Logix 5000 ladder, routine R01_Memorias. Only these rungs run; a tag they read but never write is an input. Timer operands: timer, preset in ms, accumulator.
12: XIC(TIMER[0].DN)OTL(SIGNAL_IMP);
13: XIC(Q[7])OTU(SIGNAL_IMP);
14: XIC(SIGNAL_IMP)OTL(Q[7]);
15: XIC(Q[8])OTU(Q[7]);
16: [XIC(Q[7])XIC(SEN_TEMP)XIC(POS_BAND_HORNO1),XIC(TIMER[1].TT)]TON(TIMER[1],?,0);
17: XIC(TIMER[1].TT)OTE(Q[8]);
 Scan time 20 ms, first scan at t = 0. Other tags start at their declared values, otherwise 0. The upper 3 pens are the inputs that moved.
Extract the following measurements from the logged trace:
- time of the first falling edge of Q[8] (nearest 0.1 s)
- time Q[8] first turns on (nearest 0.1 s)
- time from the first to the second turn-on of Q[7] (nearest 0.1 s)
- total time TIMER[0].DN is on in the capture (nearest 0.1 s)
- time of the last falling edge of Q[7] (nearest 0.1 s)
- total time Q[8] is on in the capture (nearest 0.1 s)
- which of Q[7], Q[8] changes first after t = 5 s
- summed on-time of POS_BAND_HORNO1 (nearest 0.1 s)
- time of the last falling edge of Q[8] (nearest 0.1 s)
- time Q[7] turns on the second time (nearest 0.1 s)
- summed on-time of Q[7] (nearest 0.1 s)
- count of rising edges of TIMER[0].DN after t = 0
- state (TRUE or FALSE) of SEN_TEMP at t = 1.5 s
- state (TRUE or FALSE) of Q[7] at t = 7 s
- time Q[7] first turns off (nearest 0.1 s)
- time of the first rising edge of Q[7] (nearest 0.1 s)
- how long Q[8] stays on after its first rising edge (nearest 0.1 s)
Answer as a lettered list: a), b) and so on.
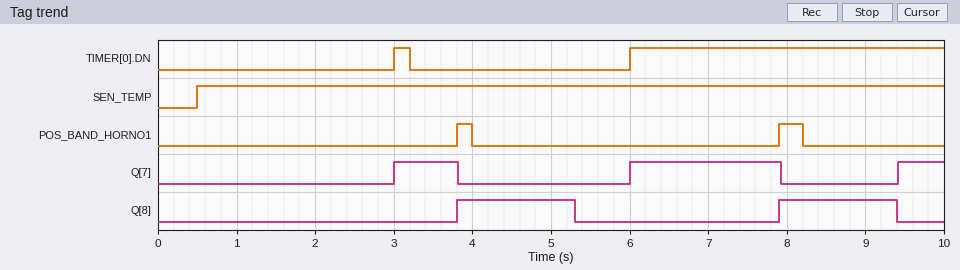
a) 5.3 s
b) 3.8 s
c) 3.0 s
d) 4.2 s
e) 7.9 s
f) 3.0 s
g) Q[8]
h) 0.5 s
i) 9.4 s
j) 6.0 s
k) 3.3 s
l) 2
m) TRUE
n) TRUE
o) 3.8 s
p) 3.0 s
q) 1.5 s
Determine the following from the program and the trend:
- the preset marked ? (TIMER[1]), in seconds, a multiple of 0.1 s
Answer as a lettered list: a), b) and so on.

a) 1.5 s
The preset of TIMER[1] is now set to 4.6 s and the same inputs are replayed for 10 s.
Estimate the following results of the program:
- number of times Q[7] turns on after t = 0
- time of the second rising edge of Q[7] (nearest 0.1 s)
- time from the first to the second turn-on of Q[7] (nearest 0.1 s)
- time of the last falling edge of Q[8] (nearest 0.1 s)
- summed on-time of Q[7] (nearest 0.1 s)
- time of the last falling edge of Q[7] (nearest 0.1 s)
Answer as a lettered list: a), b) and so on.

a) 2
b) 8.4 s
c) 5.4 s
d) 8.4 s
e) 2.4 s
f) 3.8 s
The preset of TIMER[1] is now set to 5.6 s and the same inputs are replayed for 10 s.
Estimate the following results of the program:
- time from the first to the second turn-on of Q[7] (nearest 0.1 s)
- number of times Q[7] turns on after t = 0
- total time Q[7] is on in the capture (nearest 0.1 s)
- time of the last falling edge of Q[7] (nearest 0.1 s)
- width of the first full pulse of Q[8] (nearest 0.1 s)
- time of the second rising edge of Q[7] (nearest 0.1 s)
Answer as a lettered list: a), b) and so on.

a) 6.4 s
b) 2
c) 1.4 s
d) 3.8 s
e) 5.6 s
f) 9.4 s
